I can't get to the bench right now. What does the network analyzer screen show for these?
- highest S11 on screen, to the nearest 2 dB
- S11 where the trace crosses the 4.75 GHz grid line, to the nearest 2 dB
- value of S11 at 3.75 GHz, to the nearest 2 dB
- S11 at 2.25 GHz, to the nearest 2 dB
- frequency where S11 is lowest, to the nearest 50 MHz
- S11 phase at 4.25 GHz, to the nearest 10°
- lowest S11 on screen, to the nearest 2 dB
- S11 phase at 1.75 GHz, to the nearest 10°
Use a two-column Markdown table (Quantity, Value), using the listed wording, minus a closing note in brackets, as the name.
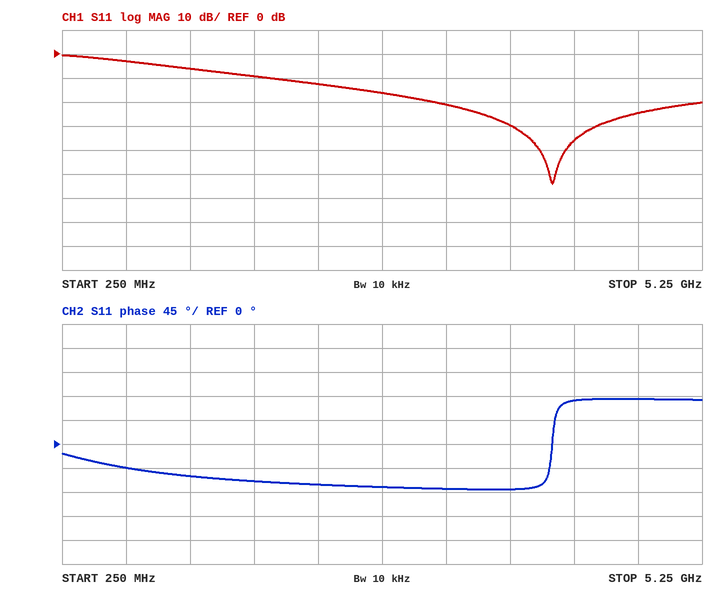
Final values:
| Quantity | Value |
|---|---|
| highest S11 on screen, to the nearest 2 dB | 0 dB |
| S11 where the trace crosses the 4.75 GHz grid line, to the nearest 2 dB | -24 dB |
| value of S11 at 3.75 GHz, to the nearest 2 dB | -30 dB |
| S11 at 2.25 GHz, to the nearest 2 dB | -12 dB |
| frequency where S11 is lowest, to the nearest 50 MHz | 4.10 GHz |
| S11 phase at 4.25 GHz, to the nearest 10° | 80° |
| lowest S11 on screen, to the nearest 2 dB | -54 dB |
| S11 phase at 1.75 GHz, to the nearest 10° | -70° |
